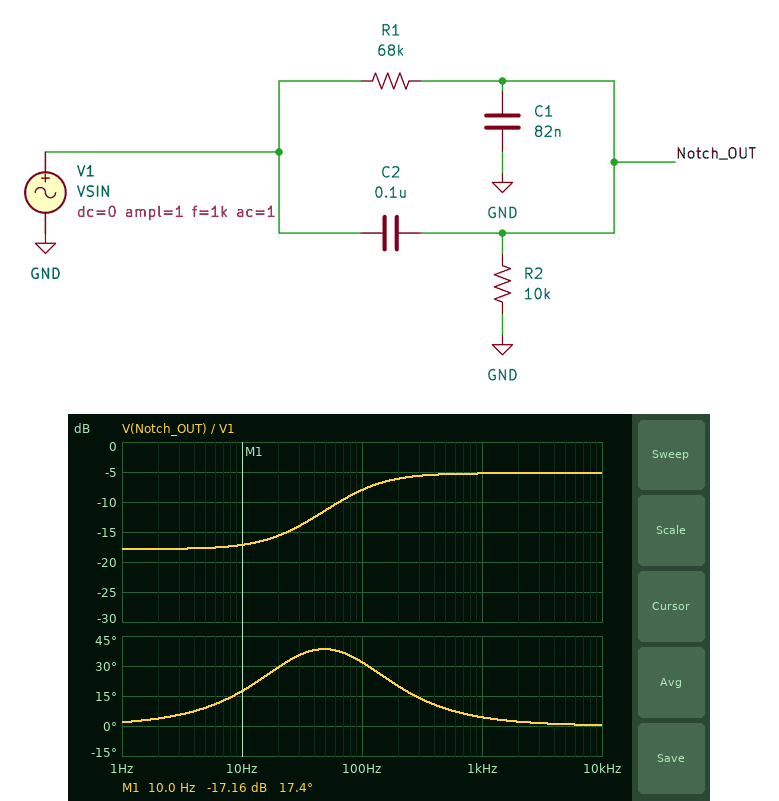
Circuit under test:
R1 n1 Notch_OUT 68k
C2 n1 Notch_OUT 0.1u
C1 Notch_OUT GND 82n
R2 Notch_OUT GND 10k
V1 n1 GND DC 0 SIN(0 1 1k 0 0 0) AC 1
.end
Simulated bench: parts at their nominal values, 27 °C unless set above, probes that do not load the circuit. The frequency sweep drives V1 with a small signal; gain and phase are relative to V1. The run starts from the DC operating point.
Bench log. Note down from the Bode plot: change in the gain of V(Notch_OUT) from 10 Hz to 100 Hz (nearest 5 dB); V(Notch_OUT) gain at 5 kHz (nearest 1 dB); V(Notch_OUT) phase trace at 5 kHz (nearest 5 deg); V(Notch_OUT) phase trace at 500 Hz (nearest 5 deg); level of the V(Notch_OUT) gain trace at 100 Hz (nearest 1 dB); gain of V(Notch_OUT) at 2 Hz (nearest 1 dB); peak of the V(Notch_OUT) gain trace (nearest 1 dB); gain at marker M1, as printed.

10 dB
-5 dB
0 deg
10 deg
-8 dB
-18 dB
-5 dB
-17.16 dB
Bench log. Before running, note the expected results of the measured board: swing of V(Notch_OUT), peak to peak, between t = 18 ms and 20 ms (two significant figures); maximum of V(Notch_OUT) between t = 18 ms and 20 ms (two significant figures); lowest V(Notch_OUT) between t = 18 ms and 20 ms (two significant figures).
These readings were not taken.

1.1 V
550 mV
-550 mV
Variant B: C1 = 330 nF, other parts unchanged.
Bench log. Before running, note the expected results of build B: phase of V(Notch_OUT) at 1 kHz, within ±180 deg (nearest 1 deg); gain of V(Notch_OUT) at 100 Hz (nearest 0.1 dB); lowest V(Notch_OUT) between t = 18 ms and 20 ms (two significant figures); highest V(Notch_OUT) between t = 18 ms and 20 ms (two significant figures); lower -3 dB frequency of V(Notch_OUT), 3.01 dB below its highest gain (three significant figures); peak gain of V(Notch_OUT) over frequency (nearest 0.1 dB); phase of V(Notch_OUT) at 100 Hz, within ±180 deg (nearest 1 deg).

1 deg
-13.2 dB
-230 mV
230 mV
26.6 Hz
-12.7 dB
10 deg
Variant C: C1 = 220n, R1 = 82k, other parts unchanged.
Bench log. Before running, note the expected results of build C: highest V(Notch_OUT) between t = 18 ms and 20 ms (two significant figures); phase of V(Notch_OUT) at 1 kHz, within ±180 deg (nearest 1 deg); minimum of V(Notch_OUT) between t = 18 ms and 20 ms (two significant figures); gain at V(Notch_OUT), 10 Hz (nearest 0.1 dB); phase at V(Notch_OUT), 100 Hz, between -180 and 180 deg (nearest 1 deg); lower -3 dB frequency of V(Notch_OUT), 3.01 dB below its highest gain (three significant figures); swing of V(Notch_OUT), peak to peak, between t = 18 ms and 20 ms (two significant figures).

310 mV
2 deg
-310 mV
-18.4 dB
18 deg
48.6 Hz
620 mV
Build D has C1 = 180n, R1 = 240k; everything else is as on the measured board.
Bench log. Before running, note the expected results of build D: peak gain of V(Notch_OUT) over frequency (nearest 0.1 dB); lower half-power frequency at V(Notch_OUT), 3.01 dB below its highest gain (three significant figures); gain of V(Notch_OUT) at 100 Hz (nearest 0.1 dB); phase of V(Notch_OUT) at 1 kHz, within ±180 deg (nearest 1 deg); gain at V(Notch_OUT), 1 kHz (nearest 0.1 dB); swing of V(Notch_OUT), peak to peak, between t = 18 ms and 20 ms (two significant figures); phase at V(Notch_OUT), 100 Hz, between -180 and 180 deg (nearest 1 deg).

-8.9 dB
58.5 Hz
-10.2 dB
3 deg
-9.0 dB
710 mV
27 deg
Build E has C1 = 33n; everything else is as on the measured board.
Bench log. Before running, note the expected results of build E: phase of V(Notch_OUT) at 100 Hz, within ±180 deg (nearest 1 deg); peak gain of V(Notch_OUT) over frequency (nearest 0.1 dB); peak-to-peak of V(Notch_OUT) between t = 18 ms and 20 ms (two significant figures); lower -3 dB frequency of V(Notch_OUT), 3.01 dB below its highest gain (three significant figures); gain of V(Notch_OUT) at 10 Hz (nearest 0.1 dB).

41 deg
-2.5 dB
1.5 V
133 Hz
-17.1 dB
